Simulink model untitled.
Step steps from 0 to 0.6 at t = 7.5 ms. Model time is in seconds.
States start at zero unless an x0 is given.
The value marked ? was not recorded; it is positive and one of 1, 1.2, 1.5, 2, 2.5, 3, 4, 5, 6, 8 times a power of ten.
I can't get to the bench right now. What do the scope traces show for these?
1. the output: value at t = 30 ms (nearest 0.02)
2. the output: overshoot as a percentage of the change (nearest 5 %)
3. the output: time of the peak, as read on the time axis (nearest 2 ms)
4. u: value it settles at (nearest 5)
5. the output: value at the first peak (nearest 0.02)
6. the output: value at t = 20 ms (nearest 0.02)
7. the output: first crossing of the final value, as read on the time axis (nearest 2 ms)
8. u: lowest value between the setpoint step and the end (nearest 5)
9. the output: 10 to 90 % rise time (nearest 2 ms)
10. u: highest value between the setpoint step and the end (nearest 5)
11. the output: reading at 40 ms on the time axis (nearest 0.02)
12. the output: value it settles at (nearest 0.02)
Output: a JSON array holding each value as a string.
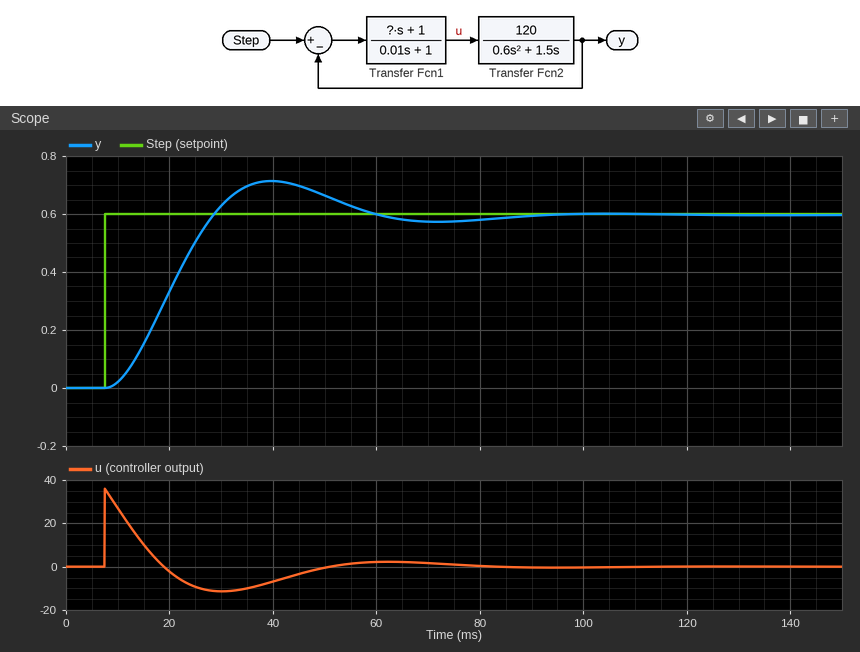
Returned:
["0.62", "20 %", "40 ms", "0", "0.72", "0.34", "28 ms", "-10", "14 ms", "35", "0.72", "0.60"]
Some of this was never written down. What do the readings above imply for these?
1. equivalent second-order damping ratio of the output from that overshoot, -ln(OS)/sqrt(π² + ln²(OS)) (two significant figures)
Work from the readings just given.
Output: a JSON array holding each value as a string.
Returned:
["0.46"]
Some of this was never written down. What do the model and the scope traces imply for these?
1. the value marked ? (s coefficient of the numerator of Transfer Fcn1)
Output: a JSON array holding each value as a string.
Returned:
["0.6"]
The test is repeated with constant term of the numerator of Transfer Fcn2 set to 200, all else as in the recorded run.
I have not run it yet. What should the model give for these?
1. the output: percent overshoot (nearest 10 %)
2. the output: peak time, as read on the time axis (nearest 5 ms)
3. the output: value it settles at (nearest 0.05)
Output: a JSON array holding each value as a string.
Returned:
["30 %", "30 ms", "0.60"]
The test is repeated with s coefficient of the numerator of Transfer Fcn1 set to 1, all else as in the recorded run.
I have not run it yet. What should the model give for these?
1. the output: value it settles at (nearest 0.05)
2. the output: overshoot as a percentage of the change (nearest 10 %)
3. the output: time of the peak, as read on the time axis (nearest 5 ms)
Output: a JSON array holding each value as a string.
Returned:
["0.60", "30 %", "30 ms"]
